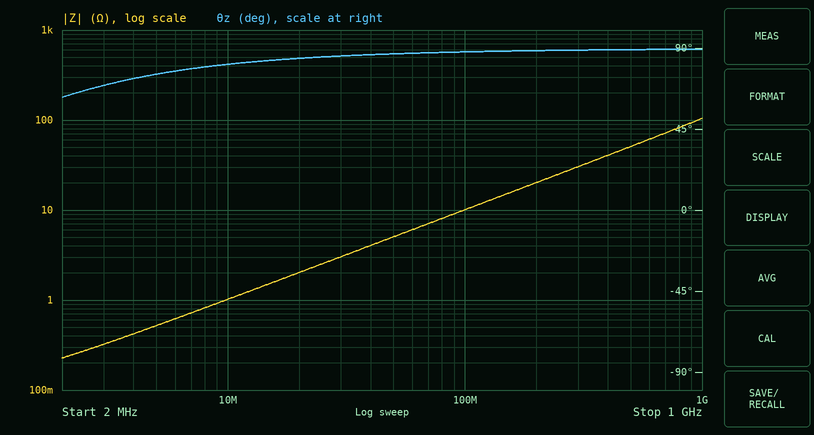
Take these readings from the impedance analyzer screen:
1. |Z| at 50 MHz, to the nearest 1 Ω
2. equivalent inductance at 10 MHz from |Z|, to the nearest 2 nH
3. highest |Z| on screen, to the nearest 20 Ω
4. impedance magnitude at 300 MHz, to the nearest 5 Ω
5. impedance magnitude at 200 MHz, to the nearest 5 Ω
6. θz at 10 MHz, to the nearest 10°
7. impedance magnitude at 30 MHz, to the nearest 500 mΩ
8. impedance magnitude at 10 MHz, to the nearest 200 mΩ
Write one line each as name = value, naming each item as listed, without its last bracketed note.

|Z| at 50 MHz, to the nearest 1 Ω = 5 Ω
equivalent inductance at 10 MHz from |Z|, to the nearest 2 nH = 16 nH
highest |Z| on screen, to the nearest 20 Ω = 100 Ω
impedance magnitude at 300 MHz, to the nearest 5 Ω = 30 Ω
impedance magnitude at 200 MHz, to the nearest 5 Ω = 20 Ω
θz at 10 MHz, to the nearest 10° = 80°
impedance magnitude at 30 MHz, to the nearest 500 mΩ = 3.0 Ω
impedance magnitude at 10 MHz, to the nearest 200 mΩ = 1.0 Ω
